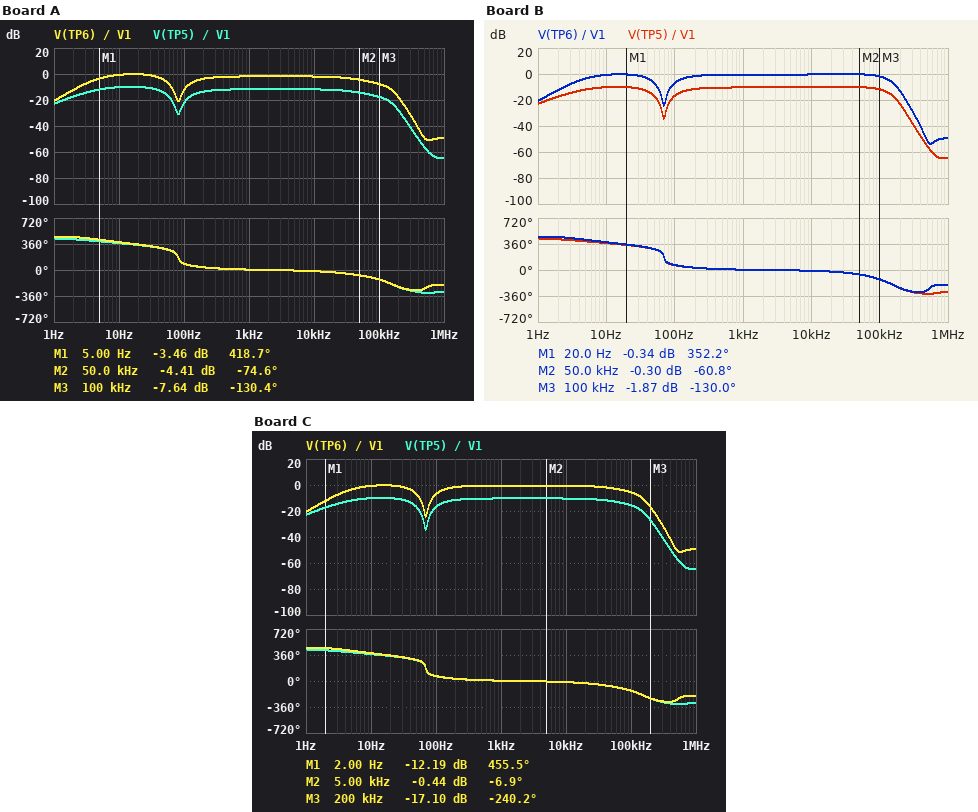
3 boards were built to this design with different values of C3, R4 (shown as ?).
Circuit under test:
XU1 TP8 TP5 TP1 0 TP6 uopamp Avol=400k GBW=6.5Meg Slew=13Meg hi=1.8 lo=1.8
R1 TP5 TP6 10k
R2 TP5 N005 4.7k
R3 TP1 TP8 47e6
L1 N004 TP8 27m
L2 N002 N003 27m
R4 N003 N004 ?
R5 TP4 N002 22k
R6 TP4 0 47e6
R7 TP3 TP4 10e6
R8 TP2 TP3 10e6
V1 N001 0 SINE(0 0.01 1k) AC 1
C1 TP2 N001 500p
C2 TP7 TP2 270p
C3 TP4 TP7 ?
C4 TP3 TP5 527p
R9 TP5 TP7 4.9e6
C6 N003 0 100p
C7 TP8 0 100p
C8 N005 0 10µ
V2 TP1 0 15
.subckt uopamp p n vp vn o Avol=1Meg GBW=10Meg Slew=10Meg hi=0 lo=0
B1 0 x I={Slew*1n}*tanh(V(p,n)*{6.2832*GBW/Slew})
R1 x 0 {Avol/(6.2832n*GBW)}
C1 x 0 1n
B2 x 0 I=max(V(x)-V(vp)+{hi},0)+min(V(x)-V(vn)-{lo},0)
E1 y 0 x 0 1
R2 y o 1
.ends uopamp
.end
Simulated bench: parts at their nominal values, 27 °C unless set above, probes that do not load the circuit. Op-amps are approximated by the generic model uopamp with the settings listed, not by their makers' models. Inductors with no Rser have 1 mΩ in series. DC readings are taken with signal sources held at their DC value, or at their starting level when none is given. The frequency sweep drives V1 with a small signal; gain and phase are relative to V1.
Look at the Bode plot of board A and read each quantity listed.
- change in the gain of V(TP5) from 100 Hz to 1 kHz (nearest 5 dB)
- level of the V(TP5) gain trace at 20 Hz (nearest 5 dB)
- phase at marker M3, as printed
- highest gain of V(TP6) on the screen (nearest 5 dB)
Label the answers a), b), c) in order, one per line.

a) 10 dB
b) -10 dB
c) -130.4 deg
d) 0 dB
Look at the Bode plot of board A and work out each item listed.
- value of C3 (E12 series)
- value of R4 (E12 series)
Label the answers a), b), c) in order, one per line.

a) 120 pF
b) 56 kΩ
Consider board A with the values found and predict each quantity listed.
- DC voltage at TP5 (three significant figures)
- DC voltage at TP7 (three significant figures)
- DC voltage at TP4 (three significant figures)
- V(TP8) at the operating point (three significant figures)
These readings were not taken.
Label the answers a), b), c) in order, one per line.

a) 7.51 V
b) 7.51 V
c) 7.49 V
d) 7.51 V
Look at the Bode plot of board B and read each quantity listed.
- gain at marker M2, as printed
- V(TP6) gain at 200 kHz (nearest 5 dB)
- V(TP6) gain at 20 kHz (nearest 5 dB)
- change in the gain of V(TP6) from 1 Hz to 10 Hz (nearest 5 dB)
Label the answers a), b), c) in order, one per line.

a) -0.30 dB
b) -15 dB
c) 0 dB
d) 20 dB
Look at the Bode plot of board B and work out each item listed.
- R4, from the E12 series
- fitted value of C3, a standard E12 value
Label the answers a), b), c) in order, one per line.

a) 27 kΩ
b) 180 pF
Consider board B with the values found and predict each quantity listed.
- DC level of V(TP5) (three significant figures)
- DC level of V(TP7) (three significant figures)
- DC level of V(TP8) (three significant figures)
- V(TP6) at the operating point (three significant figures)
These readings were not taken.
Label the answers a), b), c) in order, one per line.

a) 7.50 V
b) 7.50 V
c) 7.50 V
d) 7.50 V
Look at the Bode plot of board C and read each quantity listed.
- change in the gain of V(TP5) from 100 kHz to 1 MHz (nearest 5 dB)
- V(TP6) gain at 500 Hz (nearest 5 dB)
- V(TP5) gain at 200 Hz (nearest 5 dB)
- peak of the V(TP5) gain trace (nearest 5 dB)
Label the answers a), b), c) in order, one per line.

a) -50 dB
b) 0 dB
c) -10 dB
d) -10 dB
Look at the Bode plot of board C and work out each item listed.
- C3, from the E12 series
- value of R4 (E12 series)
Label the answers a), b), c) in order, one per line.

a) 180 pF
b) 47 kΩ
